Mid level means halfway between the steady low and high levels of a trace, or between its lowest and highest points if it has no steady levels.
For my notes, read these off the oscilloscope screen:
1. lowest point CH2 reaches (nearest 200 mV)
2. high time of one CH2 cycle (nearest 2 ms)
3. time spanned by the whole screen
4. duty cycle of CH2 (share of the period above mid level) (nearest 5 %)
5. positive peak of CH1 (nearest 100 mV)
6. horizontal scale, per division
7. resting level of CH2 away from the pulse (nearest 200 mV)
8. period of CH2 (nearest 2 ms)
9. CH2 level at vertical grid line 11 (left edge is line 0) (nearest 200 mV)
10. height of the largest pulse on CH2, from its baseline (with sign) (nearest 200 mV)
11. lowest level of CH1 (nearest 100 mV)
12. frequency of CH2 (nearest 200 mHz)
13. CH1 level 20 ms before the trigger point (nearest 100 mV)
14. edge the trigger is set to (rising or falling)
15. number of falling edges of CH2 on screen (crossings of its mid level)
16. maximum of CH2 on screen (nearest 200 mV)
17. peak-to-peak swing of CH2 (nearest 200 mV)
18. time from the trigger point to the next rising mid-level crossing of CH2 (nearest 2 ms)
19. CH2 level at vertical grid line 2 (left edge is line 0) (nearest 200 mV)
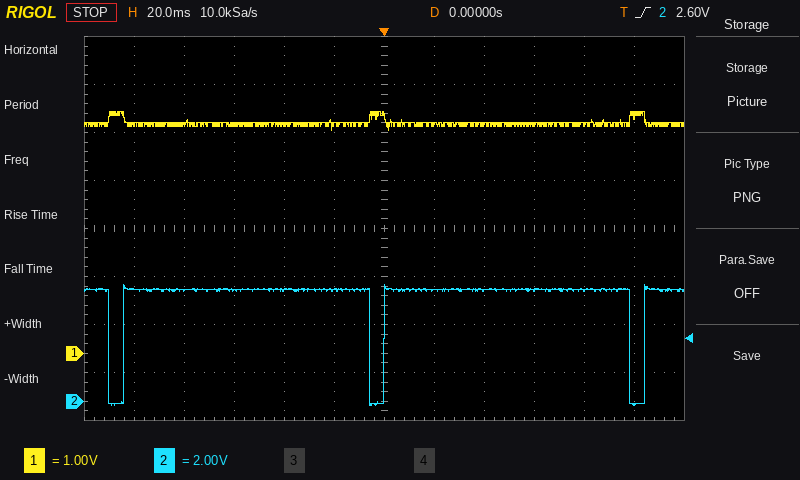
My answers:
-200 mV
98 ms
240 ms
95 %
5.0 V
20 ms
4.6 V
104 ms
-200 mV
-4.8 V
4.6 V
9.6 Hz
4.7 V
rising
3
4.8 V
5.0 V
104 ms
4.6 V
